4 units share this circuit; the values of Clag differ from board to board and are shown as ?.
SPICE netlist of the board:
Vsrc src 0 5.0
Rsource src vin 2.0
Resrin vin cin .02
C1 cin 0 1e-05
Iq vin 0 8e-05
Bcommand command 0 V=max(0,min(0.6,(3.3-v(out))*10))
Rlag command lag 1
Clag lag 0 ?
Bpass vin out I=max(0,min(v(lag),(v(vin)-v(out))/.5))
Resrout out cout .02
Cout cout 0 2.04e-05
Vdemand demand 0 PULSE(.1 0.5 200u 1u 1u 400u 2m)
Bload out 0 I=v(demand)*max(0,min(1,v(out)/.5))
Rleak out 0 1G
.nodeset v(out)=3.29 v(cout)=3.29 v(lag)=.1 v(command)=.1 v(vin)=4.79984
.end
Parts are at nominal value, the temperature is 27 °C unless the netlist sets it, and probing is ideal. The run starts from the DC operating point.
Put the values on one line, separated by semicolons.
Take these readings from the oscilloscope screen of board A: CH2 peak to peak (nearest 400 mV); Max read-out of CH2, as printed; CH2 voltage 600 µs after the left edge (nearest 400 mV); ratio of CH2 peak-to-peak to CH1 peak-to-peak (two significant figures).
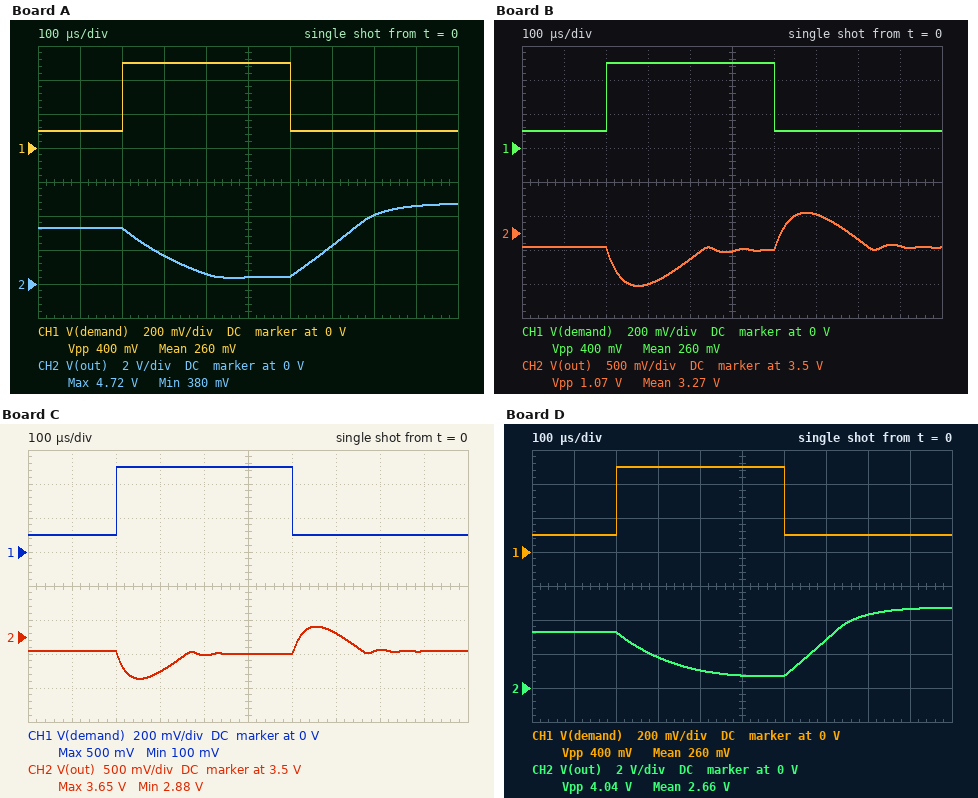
4.4 V; 4.72 V; 400 mV; 11
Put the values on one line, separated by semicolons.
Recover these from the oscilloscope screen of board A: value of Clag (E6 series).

330 µF
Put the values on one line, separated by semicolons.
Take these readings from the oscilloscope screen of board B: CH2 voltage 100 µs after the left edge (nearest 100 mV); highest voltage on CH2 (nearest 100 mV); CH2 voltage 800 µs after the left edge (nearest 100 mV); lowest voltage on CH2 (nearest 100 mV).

3.3 V; 3.8 V; 3.4 V; 2.7 V
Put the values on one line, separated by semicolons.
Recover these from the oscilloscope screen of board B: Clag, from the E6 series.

47 µF
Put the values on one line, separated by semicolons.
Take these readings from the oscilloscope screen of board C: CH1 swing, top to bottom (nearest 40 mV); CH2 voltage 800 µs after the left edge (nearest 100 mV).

400 mV; 3.3 V
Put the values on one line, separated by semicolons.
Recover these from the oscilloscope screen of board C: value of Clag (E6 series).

33 µF
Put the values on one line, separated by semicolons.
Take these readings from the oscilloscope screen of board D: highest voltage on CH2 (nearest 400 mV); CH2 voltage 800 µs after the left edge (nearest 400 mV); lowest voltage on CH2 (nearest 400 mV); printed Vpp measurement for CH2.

4.8 V; 4.4 V; 800 mV; 4.04 V
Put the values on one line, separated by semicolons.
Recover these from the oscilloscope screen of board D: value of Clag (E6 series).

220 µF
